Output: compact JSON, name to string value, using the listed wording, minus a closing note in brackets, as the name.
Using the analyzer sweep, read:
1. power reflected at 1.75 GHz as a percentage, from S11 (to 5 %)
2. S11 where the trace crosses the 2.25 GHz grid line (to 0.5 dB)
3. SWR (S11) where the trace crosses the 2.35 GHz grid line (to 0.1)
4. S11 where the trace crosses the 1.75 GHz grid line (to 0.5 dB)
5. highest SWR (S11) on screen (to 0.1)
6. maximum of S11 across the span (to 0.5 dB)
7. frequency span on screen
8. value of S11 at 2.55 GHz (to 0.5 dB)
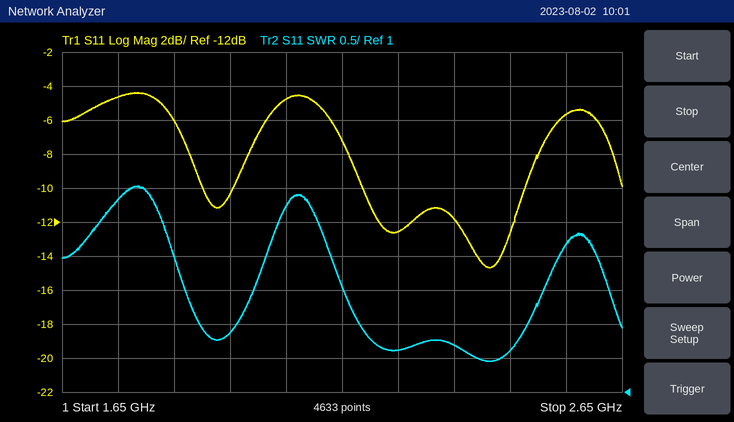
{"power reflected at 1.75 GHz as a percentage, from S11": "35 %", "S11 where the trace crosses the 2.25 GHz grid line": "-12.5 dB", "SWR (S11) where the trace crosses the 2.35 GHz grid line": "1.7", "S11 where the trace crosses the 1.75 GHz grid line": "-4.5 dB", "highest SWR (S11) on screen": "4.0", "maximum of S11 across the span": "-4.5 dB", "frequency span on screen": "1 GHz", "value of S11 at 2.55 GHz": "-5.5 dB"}
